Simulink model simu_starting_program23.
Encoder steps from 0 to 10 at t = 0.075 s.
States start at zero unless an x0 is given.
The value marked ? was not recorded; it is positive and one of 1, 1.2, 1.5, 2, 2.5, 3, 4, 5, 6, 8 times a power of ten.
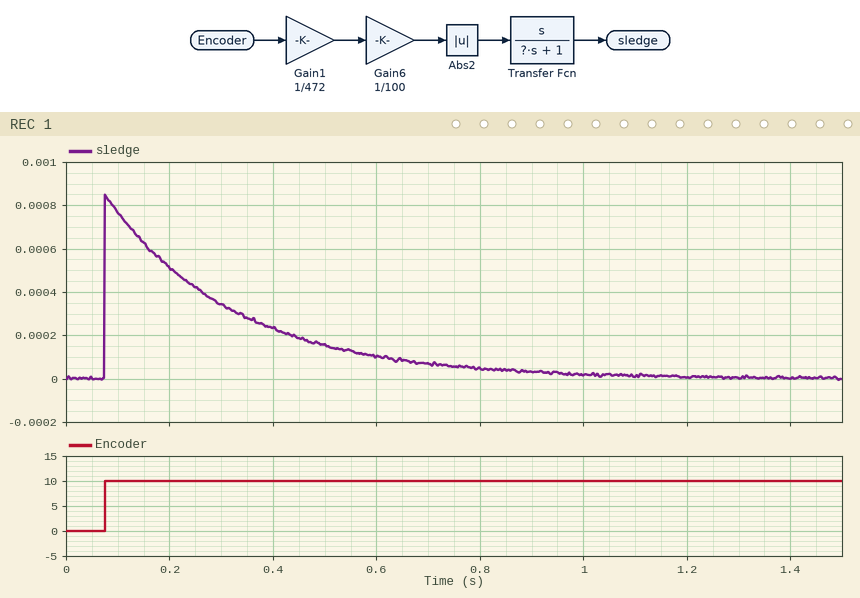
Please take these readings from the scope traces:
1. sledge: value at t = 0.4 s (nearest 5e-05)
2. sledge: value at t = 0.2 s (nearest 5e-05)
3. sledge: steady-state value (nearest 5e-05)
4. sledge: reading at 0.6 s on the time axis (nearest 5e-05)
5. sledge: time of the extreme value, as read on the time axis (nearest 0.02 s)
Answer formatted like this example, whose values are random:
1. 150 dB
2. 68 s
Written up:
1. 0.00025
2. 0.00050
3. 0.00000
4. 0.00010
5. 0.08 s
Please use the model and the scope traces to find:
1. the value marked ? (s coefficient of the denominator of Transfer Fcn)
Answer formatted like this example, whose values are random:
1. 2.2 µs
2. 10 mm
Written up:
1. 0.25
